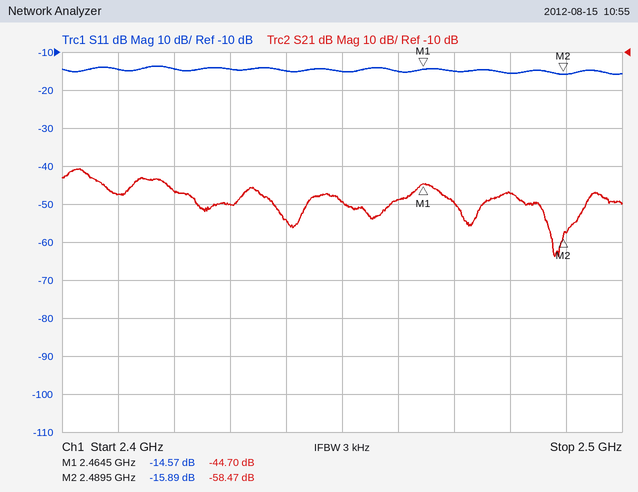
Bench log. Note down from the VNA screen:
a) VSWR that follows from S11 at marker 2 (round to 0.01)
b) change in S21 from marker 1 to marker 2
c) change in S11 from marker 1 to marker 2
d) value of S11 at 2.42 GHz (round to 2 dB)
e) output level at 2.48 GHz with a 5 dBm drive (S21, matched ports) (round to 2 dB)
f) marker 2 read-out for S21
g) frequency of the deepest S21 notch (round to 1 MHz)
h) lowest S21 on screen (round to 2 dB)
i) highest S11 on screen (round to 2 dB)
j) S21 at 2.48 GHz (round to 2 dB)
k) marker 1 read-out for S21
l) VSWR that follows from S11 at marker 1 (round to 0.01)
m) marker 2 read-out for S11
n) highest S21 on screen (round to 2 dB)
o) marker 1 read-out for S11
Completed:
1.38
-13.77 dB
-1.32 dB
-14 dB
-42 dBm
-58.47 dB
2.488 GHz
-64 dB
-14 dB
-48 dB
-44.70 dB
1.46
-15.89 dB
-40 dB
-14.57 dB
